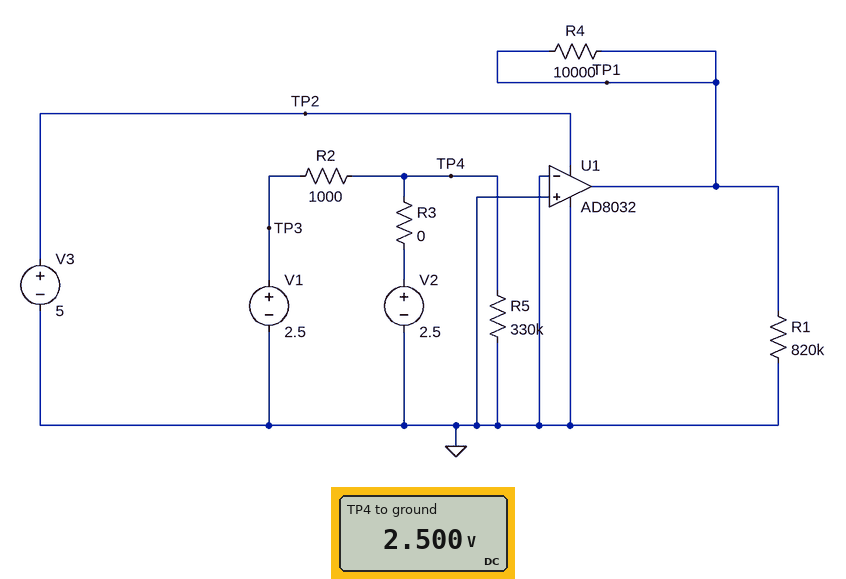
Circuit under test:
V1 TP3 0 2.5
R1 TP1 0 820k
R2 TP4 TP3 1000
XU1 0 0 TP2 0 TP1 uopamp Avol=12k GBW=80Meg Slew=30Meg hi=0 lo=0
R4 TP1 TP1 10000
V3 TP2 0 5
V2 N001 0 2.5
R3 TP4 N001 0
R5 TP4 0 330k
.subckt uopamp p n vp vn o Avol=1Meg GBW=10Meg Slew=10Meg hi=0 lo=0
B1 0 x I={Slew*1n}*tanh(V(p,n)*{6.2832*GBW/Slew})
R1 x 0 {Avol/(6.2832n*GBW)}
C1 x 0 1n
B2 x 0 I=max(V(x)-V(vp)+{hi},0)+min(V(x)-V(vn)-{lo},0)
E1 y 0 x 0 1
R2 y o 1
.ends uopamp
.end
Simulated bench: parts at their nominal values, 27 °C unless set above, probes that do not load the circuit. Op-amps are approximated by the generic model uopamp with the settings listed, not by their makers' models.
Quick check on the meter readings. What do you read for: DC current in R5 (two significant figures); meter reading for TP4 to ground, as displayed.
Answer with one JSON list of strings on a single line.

["7.6 µA", "2.500 V"]
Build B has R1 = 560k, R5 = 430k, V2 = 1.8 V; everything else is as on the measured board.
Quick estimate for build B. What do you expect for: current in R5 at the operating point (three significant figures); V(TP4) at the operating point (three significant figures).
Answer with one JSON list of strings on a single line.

["4.19 µA", "1.80 V"]
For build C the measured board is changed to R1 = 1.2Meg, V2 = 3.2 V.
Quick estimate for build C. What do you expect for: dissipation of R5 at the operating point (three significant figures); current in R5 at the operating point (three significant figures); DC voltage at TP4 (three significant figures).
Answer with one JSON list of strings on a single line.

["31.0 µW", "9.70 µA", "3.20 V"]
